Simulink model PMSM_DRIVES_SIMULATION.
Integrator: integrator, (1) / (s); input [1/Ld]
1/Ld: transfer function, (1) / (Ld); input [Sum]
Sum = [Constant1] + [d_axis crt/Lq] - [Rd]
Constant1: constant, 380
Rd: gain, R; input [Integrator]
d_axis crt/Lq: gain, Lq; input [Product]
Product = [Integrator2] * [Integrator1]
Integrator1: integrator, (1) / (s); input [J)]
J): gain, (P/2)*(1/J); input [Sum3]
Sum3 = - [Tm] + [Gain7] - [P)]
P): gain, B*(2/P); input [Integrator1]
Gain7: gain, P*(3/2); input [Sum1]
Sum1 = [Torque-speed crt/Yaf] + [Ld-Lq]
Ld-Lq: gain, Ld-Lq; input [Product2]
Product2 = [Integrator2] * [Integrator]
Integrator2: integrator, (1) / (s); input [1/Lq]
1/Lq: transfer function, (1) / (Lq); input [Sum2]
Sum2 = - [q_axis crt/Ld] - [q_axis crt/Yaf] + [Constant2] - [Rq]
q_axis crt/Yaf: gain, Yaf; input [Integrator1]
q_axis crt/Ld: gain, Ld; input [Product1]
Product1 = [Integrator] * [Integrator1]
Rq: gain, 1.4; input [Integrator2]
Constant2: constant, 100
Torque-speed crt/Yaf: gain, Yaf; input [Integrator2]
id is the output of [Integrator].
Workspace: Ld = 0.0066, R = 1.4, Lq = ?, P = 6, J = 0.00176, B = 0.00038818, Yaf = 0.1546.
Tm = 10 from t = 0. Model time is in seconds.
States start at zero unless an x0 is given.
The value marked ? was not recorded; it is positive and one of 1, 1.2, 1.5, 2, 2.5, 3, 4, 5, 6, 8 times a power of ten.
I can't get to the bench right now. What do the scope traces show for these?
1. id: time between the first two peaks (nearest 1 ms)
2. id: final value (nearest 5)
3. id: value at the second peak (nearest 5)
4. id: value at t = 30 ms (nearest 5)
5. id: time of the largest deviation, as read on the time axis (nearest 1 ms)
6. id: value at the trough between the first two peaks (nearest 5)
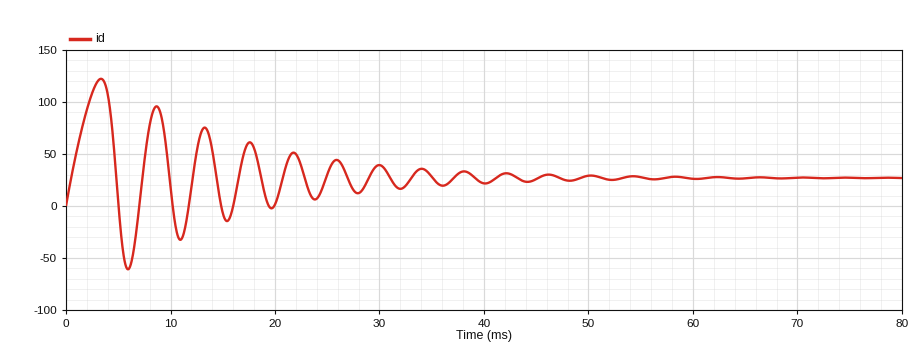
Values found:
5 ms
25
95
40
3 ms
-60
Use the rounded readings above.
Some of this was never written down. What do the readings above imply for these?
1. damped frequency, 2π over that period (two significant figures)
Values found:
1.3 rad/ms
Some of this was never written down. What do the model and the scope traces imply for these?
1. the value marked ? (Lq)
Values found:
0.012
